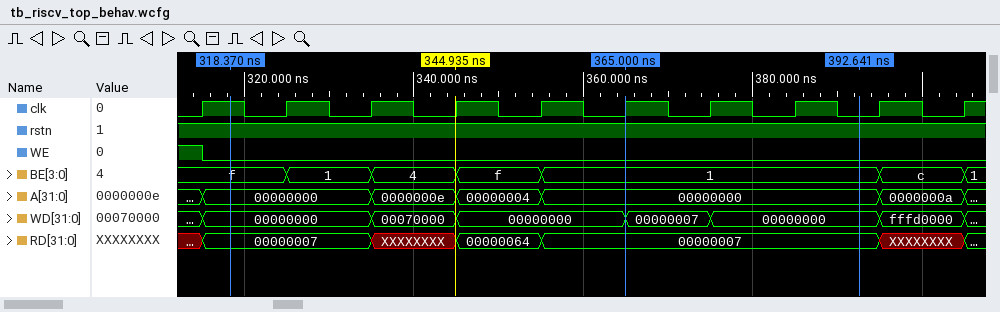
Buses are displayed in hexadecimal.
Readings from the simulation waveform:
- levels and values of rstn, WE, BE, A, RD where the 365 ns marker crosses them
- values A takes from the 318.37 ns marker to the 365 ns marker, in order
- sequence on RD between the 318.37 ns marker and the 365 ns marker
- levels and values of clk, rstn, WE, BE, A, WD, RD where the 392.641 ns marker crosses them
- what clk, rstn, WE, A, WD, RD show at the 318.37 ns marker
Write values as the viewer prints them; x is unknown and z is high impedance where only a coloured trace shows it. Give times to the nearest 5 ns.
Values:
rstn=1, WE=0, BE=1, A=00000000, RD=00000007
00000000, 0000000e, 00000004, 00000000
00000007, XXXXXXXX, 00000064, 00000007
clk=0, rstn=1, WE=0, BE=1, A=00000000, WD=00000000, RD=00000007
clk=1, rstn=1, WE=0, A=00000000, WD=00000000, RD=00000007
